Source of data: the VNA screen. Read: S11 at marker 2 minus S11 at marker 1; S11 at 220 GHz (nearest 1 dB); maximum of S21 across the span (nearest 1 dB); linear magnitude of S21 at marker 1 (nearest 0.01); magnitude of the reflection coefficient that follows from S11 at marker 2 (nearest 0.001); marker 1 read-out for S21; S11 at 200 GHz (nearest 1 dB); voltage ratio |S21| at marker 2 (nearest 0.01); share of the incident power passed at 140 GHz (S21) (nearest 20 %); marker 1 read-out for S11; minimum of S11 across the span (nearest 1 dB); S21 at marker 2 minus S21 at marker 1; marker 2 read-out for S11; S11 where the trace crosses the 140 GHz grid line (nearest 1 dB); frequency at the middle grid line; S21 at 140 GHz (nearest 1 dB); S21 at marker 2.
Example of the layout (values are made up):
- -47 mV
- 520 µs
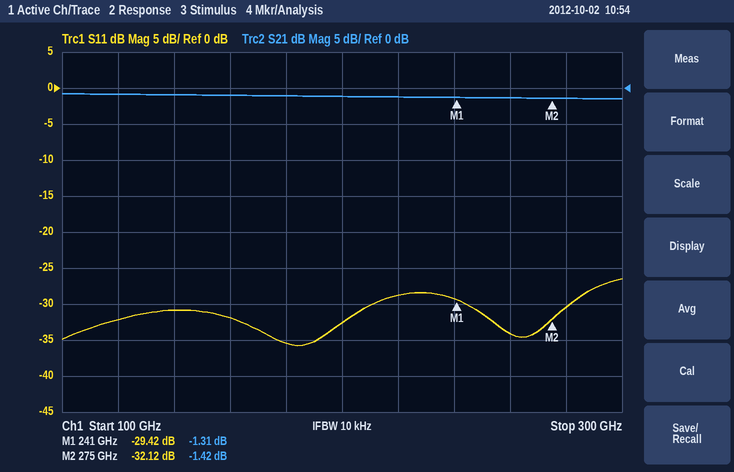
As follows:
- -2.70 dB
- -29 dB
- -1 dB
- 0.86
- 0.025
- -1.31 dB
- -33 dB
- 0.85
- 80 %
- -29.42 dB
- -36 dB
- -0.11 dB
- -32.12 dB
- -31 dB
- 200 GHz
- -1 dB
- -1.42 dB
